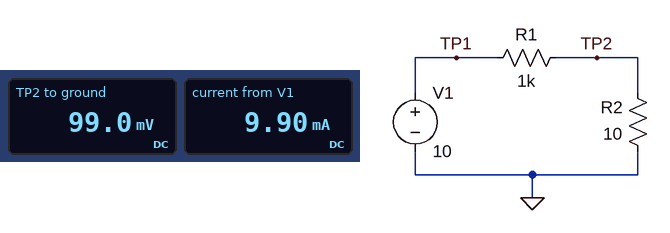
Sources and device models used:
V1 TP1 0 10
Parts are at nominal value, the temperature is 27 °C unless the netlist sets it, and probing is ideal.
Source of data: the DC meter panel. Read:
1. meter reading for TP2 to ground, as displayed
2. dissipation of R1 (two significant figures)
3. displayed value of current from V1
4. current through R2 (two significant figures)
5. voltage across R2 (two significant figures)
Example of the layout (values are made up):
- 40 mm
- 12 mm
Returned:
- 99.0 mV
- 98 mW
- 9.90 mA
- 9.9 mA
- 99 mV
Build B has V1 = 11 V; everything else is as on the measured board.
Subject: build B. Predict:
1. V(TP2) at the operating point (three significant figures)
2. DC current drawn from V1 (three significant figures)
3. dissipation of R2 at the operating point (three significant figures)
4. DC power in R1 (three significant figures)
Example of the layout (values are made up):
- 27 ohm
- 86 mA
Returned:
- 109 mV
- 10.9 mA
- 1.19 mW
- 119 mW
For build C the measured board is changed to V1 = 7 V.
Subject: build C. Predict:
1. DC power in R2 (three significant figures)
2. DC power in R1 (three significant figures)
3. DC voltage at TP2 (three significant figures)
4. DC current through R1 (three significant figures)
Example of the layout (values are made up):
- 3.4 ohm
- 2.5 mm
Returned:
- 480 µW
- 48.0 mW
- 69.3 mV
- 6.93 mA
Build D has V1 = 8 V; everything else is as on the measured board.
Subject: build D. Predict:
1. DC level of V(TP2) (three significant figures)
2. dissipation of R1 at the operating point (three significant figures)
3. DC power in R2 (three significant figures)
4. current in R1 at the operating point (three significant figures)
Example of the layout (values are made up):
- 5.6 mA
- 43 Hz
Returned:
- 79.2 mV
- 62.7 mW
- 627 µW
- 7.92 mA
